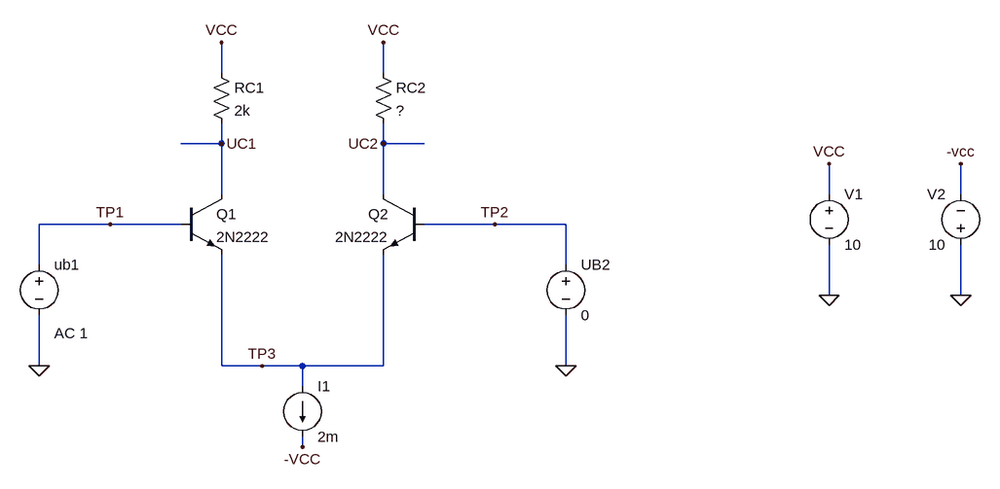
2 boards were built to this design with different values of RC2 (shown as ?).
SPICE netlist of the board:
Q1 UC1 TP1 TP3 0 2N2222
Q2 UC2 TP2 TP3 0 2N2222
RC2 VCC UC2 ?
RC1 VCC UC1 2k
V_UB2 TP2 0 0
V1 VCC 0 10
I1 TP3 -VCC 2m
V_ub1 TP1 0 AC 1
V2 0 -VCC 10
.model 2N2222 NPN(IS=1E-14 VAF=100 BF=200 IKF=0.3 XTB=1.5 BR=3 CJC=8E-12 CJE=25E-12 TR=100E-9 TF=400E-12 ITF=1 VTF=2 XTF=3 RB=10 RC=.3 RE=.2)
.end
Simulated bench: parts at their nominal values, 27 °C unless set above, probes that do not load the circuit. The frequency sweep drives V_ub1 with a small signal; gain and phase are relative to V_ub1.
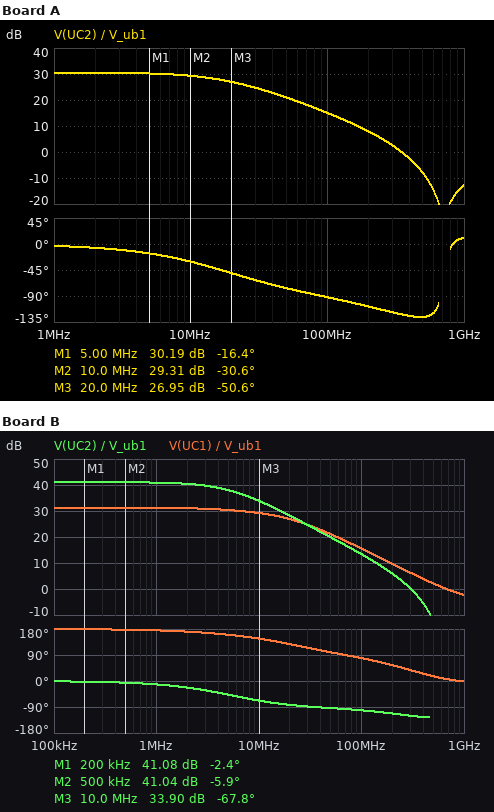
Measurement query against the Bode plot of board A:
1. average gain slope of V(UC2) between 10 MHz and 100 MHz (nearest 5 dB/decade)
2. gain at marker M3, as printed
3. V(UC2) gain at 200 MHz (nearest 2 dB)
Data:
-15 dB/decade
26.95 dB
8 dB
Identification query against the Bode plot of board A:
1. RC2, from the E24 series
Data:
1.8 kΩ
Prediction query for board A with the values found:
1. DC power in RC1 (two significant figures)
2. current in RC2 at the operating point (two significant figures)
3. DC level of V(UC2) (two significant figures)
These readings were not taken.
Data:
2.0 mW
1.0 mA
8.2 V
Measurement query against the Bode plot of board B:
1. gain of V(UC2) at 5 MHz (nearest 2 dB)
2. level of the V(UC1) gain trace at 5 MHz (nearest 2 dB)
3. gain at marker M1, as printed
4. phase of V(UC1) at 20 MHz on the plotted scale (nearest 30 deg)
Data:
38 dB
30 dB
41.08 dB
120 deg
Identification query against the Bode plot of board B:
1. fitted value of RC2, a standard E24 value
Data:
6.2 kΩ
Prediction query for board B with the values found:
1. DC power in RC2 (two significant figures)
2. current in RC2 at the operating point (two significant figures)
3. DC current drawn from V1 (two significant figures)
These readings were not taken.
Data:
5.9 mW
980 µA
2.0 mA
